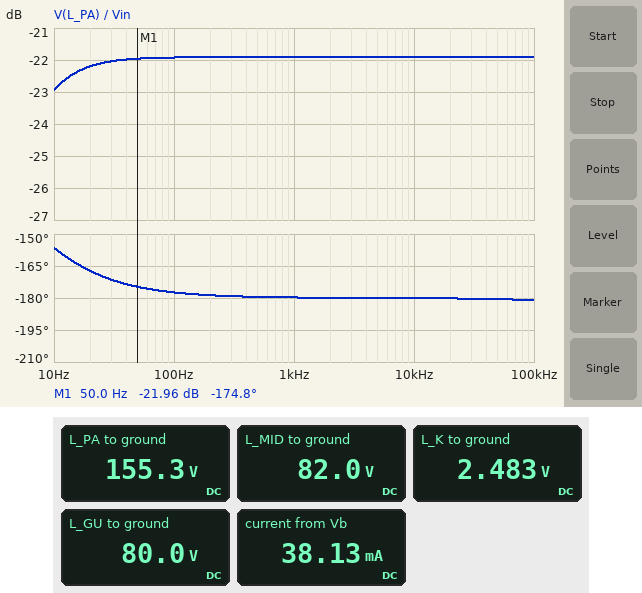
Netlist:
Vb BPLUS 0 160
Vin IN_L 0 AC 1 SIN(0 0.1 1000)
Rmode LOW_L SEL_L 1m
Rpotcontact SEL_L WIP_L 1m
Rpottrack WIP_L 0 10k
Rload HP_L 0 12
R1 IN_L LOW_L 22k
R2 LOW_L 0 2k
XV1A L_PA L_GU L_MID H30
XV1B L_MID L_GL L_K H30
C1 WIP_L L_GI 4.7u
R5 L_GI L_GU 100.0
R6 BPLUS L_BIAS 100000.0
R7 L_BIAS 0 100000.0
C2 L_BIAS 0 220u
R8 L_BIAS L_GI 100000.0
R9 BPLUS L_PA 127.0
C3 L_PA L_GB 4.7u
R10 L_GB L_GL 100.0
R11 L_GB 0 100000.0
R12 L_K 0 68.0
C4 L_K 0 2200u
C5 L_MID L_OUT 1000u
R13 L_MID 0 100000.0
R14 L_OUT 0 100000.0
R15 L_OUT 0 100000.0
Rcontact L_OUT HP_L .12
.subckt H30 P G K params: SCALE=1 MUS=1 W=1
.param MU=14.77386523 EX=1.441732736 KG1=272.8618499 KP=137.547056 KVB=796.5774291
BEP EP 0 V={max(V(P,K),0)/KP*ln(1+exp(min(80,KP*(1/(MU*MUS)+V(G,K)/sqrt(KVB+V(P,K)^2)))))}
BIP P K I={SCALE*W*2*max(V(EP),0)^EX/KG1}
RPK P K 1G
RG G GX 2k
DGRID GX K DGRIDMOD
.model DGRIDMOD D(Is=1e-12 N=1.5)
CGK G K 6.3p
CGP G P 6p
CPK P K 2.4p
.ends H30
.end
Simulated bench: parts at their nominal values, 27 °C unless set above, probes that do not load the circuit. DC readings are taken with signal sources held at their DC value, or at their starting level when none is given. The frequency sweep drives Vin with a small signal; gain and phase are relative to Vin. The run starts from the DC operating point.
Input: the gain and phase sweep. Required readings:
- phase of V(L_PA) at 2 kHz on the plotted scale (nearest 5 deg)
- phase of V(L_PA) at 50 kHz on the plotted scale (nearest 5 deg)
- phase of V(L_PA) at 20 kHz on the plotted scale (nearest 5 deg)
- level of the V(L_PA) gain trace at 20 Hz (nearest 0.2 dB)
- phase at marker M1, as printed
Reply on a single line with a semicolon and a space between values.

-180 deg; -180 deg; -180 deg; -22.2 dB; -174.8 deg
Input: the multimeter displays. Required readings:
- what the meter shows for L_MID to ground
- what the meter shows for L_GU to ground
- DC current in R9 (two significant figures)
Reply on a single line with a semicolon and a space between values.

82.0 V; 80.0 V; 37 mA
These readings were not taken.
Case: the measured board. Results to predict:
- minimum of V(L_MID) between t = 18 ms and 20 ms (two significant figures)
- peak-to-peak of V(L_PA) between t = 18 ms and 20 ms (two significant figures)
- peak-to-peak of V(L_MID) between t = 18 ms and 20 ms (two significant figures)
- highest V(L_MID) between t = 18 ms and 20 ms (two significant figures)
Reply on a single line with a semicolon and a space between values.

82 V; 16 mV; 4.6 mV; 82 V
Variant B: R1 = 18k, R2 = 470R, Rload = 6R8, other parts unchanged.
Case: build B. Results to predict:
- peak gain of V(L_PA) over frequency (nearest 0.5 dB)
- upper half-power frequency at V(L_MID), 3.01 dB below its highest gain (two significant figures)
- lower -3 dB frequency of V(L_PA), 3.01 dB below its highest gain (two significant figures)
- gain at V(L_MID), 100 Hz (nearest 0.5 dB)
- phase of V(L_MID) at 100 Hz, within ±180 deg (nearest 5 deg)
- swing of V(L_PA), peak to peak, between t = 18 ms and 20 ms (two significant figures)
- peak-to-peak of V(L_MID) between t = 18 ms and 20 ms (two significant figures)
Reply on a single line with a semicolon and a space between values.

-29.5 dB; 7.1 Hz; 6.0 Hz; -45.0 dB; -10 deg; 6.6 mV; 1.1 mV
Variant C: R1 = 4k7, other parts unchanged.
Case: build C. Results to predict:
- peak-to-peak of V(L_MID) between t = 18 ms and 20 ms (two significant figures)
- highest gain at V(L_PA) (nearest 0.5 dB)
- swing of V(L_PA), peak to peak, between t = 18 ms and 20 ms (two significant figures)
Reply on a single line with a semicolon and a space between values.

17 mV; -10.5 dB; 60 mV
